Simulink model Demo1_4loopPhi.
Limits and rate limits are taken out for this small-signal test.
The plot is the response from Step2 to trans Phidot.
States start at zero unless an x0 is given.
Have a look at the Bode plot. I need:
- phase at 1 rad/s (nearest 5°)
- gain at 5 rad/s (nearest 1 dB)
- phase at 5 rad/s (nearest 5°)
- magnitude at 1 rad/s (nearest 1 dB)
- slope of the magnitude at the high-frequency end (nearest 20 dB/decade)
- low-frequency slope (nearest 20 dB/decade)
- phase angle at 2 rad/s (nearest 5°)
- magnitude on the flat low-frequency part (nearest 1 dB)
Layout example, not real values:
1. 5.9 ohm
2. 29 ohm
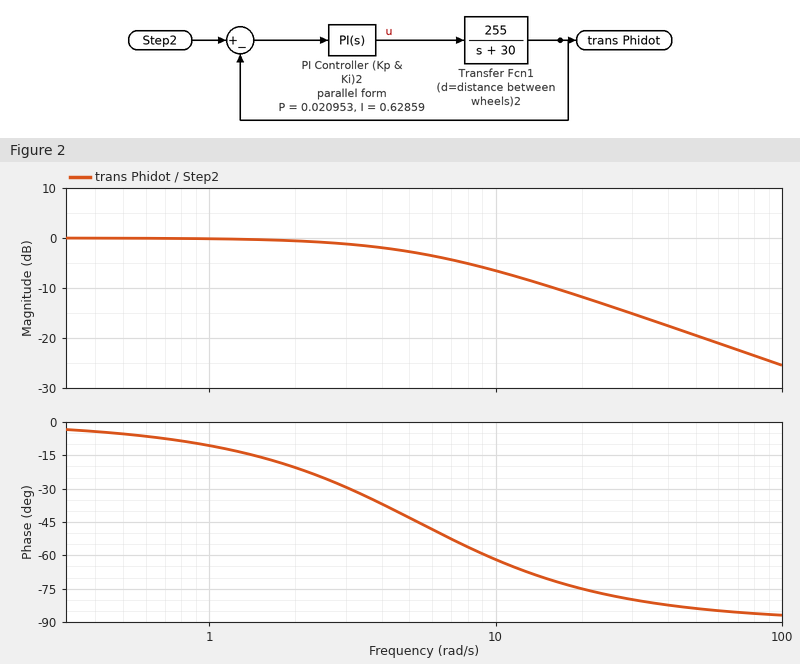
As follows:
1. -10°
2. -3 dB
3. -45°
4. 0 dB
5. -20 dB/decade
6. 0 dB/decade
7. -20°
8. 0 dB
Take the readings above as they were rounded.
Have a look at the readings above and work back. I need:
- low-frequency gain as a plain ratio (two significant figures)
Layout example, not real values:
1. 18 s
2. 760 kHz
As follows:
1. 1.0
